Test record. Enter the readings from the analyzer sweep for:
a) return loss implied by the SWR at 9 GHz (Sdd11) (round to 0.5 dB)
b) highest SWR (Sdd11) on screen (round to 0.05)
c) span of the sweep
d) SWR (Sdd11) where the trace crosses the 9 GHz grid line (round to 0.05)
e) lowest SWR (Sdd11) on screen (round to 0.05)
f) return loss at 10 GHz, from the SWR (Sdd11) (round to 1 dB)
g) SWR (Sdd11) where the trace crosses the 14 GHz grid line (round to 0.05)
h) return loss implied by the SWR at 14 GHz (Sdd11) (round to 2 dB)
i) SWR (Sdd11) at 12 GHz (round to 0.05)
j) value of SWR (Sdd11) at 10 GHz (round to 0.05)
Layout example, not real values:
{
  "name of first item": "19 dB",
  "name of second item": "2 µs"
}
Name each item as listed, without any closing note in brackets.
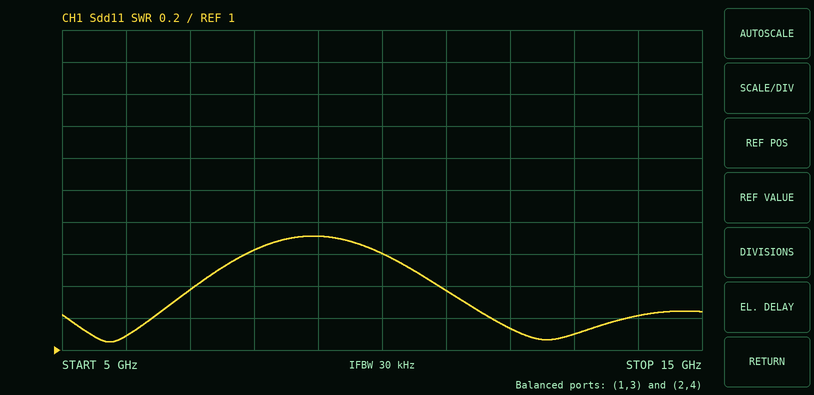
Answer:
{
  "return loss implied by the SWR at 9 GHz (Sdd11)": "11.5 dB",
  "highest SWR (Sdd11) on screen": "1.70",
  "span of the sweep": "10 GHz",
  "SWR (Sdd11) where the trace crosses the 9 GHz grid line": "1.70",
  "lowest SWR (Sdd11) on screen": "1.05",
  "return loss at 10 GHz, from the SWR (Sdd11)": "13 dB",
  "SWR (Sdd11) where the trace crosses the 14 GHz grid line": "1.20",
  "return loss implied by the SWR at 14 GHz (Sdd11)": "20 dB",
  "SWR (Sdd11) at 12 GHz": "1.15",
  "value of SWR (Sdd11) at 10 GHz": "1.60"
}
